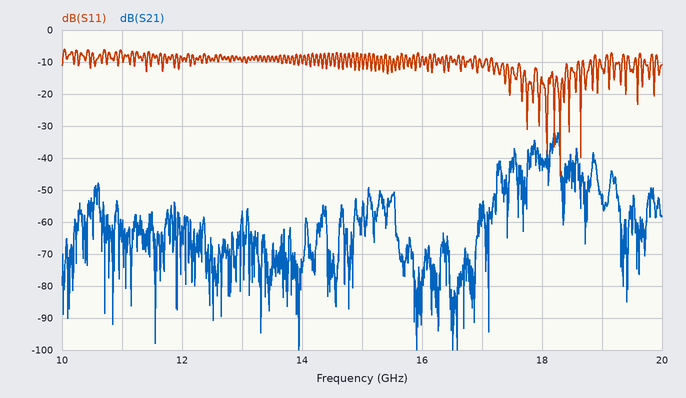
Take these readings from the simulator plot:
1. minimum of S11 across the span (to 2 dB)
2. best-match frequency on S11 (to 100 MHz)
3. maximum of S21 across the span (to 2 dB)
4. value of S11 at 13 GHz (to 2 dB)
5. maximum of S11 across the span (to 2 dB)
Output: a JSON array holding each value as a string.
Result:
["-46 dB", "18.3 GHz", "-32 dB", "-10 dB", "-6 dB"]
